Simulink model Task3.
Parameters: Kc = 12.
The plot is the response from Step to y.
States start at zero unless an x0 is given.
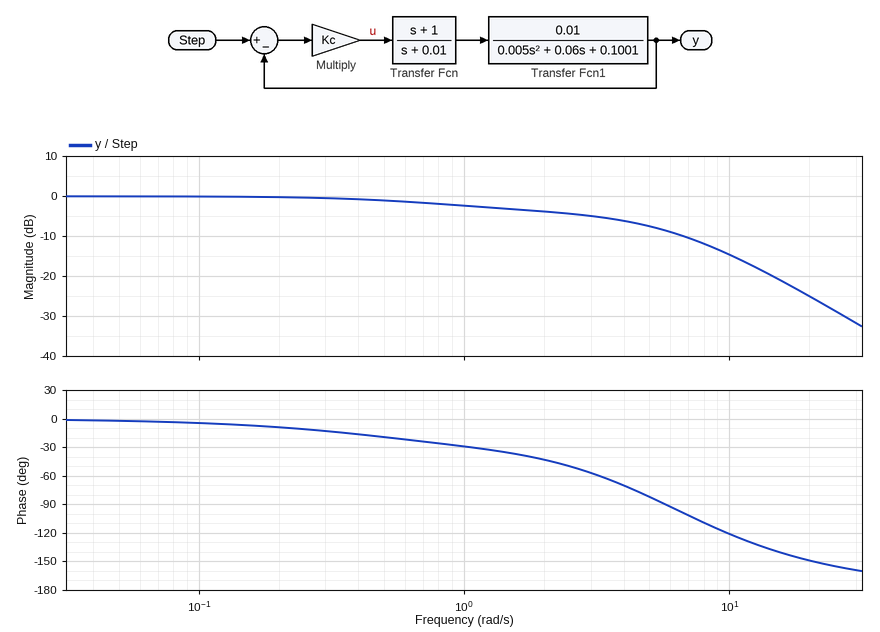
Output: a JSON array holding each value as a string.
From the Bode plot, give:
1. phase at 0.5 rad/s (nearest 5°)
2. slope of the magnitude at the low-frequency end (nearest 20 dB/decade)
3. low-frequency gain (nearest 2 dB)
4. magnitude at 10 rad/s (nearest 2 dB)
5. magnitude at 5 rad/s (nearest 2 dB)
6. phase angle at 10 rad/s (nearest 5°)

["-20°", "0 dB/decade", "0 dB", "-14 dB", "-8 dB", "-120°"]
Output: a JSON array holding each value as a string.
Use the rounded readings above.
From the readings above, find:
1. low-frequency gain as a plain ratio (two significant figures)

["1.0"]
